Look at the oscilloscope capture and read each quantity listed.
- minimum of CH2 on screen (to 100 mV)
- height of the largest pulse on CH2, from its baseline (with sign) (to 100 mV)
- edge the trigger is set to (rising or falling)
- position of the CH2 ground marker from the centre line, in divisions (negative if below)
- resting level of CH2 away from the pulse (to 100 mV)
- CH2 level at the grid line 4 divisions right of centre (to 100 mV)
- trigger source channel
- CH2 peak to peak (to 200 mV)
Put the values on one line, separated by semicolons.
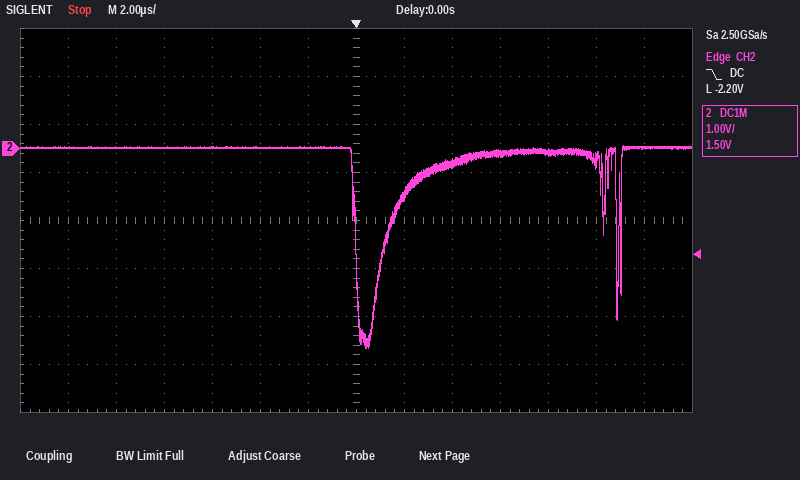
-4.2 V; -4.2 V; falling; +1.5 div; 0.0 V; -100 mV; CH2; 4.2 V
